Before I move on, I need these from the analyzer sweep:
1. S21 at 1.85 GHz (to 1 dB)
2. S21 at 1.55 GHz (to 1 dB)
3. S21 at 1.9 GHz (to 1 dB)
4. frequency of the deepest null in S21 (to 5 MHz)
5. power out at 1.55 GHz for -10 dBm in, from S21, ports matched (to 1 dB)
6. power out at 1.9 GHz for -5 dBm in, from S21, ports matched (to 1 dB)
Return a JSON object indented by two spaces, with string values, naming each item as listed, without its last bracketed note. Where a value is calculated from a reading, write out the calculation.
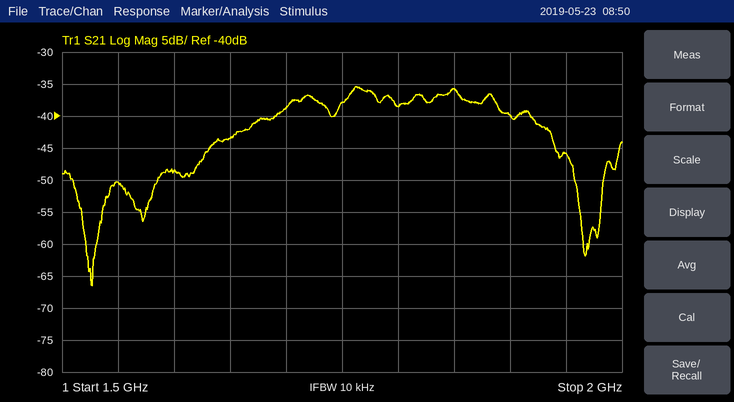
{
  "S21 at 1.85 GHz": "-36 dB",
  "S21 at 1.55 GHz": "-50 dB",
  "S21 at 1.9 GHz": "-40 dB",
  "frequency of the deepest null in S21": "1.525 GHz",
  "power out at 1.55 GHz for -10 dBm in, from S21, ports matched": "-10 dBm + (-50 dB) = -60 dBm",
  "power out at 1.9 GHz for -5 dBm in, from S21, ports matched": "-5 dBm + (-40 dB) = -45 dBm"
}
